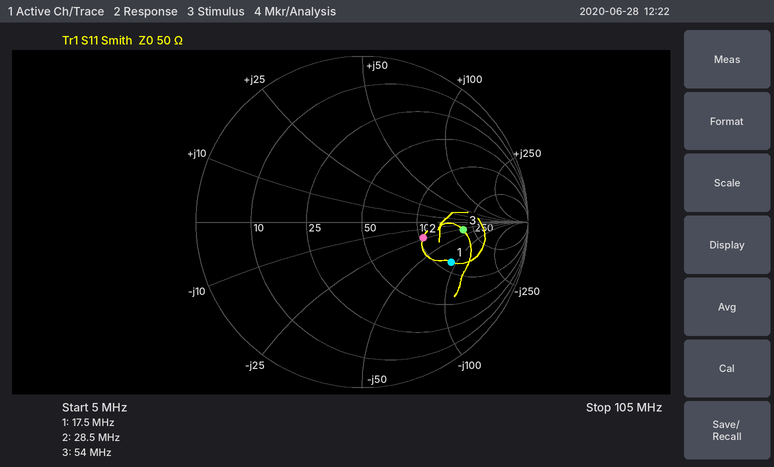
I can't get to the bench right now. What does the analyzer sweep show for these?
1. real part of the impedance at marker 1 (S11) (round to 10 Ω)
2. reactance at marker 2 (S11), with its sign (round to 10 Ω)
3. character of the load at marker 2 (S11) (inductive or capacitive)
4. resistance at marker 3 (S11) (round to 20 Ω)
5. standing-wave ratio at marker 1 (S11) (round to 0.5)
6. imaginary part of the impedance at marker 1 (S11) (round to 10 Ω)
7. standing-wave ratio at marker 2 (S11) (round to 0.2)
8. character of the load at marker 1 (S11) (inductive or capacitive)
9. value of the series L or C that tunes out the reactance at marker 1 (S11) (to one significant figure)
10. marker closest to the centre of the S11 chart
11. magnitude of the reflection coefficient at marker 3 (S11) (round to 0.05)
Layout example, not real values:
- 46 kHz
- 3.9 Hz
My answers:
- 120 Ω
- -20 Ω
- capacitive
- 200 Ω
- 4.0
- -90 Ω
- 2.2
- capacitive
- 800 nH
- marker 2
- 0.60
